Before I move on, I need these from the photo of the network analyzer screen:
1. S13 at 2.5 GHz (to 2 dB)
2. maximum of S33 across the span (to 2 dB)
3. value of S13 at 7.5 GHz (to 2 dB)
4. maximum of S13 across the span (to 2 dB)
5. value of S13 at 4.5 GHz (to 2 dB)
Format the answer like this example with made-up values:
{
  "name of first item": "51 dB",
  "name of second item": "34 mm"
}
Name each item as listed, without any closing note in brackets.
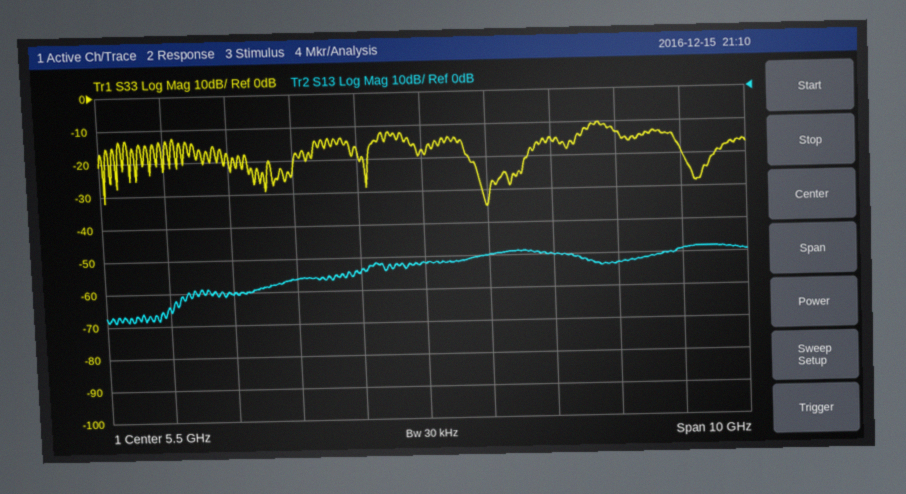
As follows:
{
  "S13 at 2.5 GHz": "-60 dB",
  "maximum of S33 across the span": "-10 dB",
  "value of S13 at 7.5 GHz": "-50 dB",
  "maximum of S13 across the span": "-48 dB",
  "value of S13 at 4.5 GHz": "-54 dB"
}
